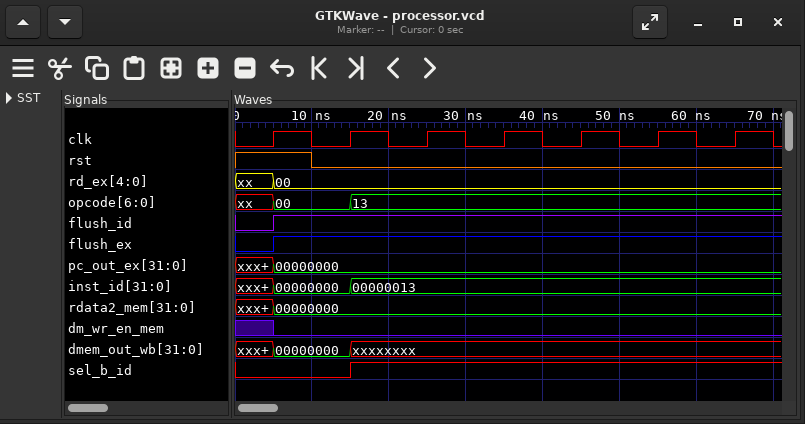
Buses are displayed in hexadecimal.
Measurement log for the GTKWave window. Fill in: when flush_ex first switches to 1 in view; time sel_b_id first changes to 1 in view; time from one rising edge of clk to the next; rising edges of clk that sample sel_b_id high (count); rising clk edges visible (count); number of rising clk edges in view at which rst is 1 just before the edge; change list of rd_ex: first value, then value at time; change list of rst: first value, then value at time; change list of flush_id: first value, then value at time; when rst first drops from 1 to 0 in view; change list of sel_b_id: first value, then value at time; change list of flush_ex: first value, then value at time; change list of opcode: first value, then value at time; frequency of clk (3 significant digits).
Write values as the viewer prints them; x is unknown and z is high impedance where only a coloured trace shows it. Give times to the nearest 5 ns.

5 ns
15 ns
10 ns
5
7
1
xx, 00 at 5 ns
1, 0 at 10 ns
0, 1 at 5 ns
10 ns
0, 1 at 15 ns
0, 1 at 5 ns
xx, 00 at 5 ns, 13 at 15 ns
100 MHz
